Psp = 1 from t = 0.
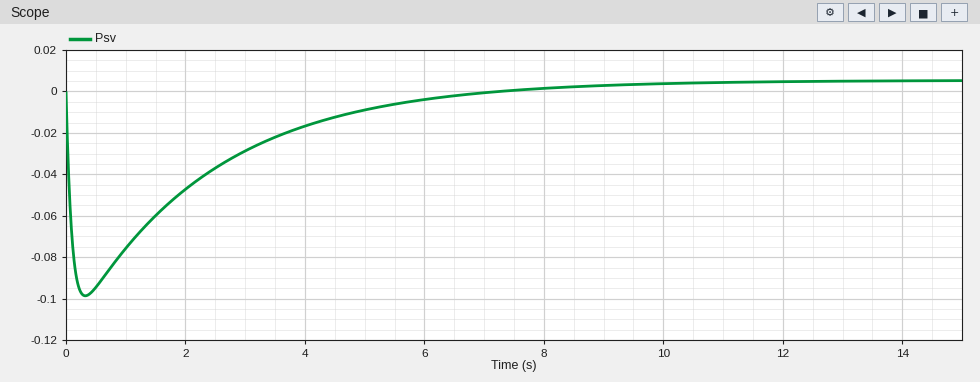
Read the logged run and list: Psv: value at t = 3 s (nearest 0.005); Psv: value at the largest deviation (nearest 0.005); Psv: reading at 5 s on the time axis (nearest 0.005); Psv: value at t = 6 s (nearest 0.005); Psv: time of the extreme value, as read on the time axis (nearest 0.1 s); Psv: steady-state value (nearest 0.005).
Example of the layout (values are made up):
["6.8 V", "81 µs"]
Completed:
["-0.030", "-0.100", "-0.010", "-0.005", "0.3 s", "0.005"]
